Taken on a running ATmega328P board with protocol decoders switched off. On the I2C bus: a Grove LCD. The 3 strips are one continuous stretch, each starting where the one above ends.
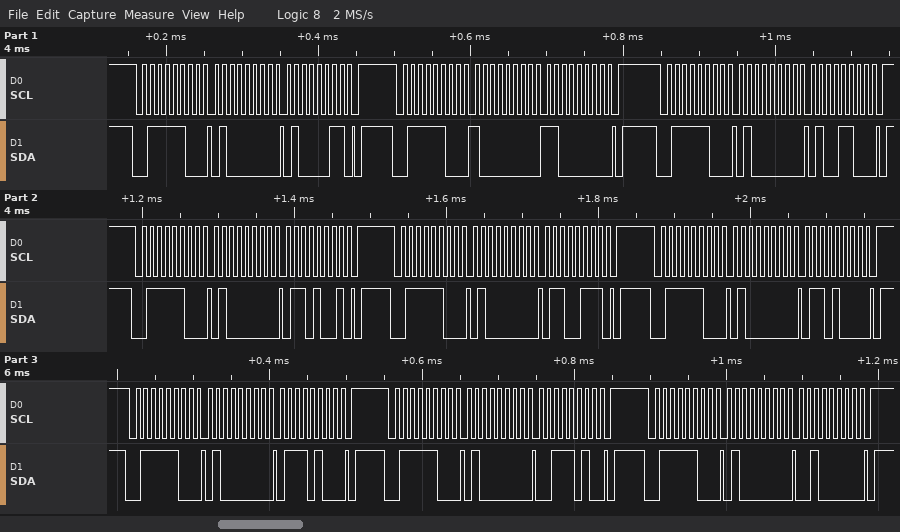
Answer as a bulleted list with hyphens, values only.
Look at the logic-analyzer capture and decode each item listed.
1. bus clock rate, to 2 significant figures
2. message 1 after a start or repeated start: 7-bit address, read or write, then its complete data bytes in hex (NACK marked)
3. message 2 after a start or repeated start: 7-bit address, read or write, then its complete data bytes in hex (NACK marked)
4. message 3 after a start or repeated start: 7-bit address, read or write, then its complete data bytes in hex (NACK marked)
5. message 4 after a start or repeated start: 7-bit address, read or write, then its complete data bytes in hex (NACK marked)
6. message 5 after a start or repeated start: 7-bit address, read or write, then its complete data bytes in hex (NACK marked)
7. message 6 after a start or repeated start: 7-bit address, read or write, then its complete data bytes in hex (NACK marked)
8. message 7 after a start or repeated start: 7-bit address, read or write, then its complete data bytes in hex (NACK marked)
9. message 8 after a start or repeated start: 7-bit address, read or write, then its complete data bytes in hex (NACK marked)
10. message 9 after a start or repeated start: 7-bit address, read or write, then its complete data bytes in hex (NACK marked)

- 100 kHz
- 0x3E write: 40 43
- 0x3E write: 80 C0
- 0x3E write: 40 4C
- 0x3E write: 40 69
- 0x3E write: 40 67
- 0x3E write: 40 68
- 0x3E write: 40 74
- 0x3E write: 40 3A
- 0x3E write: 40 20
